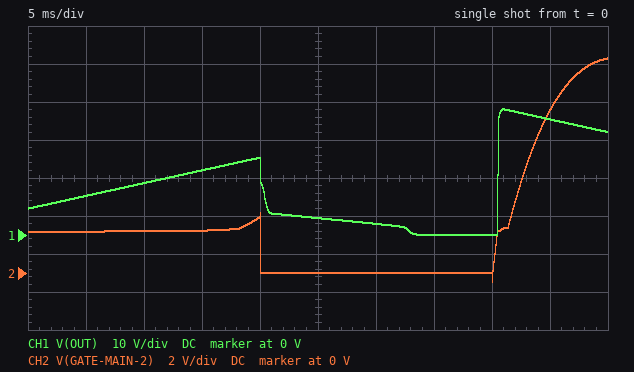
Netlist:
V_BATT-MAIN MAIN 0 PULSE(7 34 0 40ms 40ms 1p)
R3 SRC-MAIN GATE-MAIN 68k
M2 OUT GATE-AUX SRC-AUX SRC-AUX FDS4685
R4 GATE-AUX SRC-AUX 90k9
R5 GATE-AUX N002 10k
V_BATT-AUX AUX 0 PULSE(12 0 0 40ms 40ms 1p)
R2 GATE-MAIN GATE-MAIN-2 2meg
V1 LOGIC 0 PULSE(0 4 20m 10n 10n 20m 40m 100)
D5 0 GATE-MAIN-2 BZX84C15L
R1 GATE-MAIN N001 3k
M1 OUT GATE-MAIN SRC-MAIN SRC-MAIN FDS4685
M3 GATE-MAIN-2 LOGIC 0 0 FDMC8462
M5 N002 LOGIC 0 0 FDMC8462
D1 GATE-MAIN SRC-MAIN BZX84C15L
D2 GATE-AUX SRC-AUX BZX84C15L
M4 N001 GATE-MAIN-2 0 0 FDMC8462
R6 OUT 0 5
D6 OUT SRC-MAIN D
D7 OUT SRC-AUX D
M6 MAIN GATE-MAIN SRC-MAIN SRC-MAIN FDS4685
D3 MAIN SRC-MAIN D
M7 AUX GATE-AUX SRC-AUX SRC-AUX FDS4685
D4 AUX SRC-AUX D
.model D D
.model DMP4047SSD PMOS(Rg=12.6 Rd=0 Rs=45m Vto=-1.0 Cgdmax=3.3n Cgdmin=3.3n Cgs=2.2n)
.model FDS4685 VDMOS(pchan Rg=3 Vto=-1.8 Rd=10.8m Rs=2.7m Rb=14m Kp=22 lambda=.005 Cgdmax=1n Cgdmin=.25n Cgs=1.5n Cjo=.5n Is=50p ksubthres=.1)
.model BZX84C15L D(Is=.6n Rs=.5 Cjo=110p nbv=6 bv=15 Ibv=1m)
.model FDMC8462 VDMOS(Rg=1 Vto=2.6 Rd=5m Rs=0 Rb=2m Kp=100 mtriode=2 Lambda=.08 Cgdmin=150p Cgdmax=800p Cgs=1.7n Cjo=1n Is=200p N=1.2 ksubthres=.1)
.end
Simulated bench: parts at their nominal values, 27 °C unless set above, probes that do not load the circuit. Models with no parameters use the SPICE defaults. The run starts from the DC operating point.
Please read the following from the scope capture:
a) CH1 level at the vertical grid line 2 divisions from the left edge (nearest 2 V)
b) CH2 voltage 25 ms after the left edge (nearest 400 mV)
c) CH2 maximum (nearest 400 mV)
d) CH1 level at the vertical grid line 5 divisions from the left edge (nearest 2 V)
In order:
14 V
0 V
11.2 V
4 V
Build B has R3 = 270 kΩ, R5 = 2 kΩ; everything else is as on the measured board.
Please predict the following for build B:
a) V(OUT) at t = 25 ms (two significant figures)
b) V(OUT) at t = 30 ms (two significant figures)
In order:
5.4 V
4.5 V
